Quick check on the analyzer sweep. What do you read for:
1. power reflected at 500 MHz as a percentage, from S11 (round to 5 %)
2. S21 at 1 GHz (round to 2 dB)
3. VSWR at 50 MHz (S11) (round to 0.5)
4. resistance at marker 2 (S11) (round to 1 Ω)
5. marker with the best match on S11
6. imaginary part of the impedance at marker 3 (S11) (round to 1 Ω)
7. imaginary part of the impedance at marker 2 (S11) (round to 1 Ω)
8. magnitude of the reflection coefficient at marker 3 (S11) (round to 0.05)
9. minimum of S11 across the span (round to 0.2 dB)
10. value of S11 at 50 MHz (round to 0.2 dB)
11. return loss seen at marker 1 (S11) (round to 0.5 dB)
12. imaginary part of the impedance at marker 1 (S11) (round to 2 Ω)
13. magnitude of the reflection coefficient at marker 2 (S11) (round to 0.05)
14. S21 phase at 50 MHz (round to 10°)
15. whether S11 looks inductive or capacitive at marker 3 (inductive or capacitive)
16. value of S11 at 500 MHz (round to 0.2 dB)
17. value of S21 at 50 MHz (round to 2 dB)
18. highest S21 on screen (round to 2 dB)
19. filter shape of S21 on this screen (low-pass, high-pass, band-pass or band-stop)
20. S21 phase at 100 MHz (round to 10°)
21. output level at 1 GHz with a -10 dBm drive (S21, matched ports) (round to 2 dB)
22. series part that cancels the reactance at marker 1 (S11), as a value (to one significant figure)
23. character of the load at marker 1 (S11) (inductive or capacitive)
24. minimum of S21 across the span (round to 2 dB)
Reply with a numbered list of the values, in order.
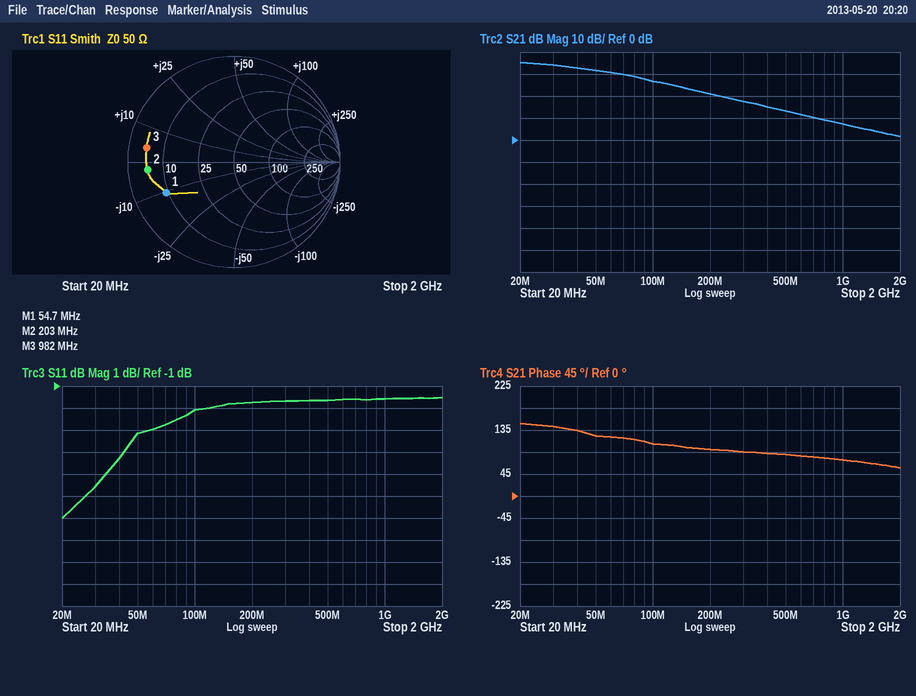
1. 70 %
2. 8 dB
3. 5.5
4. 5 Ω
5. marker 1
6. +4 Ω
7. -2 Ω
8. 0.85
9. -7.0 dB
10. -3.2 dB
11. 3.0 dB
12. -10 Ω
13. 0.80
14. 120°
15. inductive
16. -1.6 dB
17. 32 dB
18. 36 dB
19. low-pass
20. 110°
21. -2 dBm
22. 30 nH
23. capacitive
24. 2 dB
